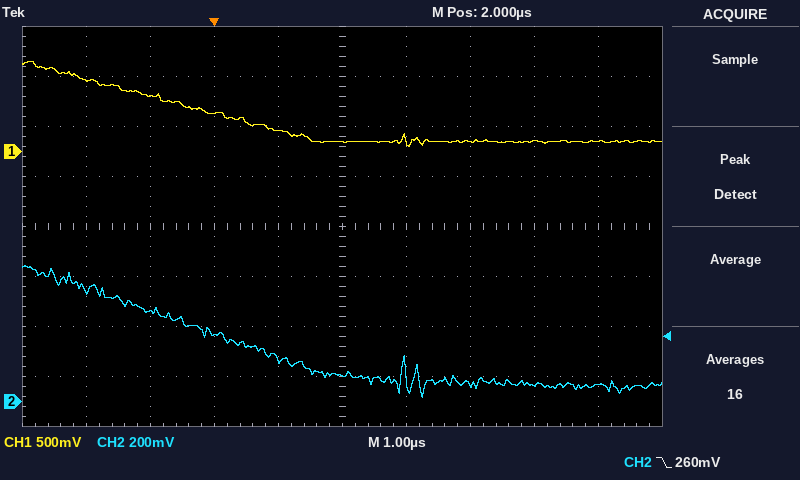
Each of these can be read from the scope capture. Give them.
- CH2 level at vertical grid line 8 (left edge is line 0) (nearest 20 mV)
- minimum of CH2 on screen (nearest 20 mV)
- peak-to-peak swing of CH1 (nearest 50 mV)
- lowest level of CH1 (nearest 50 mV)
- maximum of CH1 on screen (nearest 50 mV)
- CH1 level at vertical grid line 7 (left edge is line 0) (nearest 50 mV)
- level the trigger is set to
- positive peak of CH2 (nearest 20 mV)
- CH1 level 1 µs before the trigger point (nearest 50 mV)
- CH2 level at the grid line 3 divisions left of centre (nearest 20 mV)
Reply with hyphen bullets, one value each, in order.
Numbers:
- 60 mV
- 20 mV
- 850 mV
- 50 mV
- 900 mV
- 100 mV
- 260 mV
- 540 mV
- 550 mV
- 360 mV
